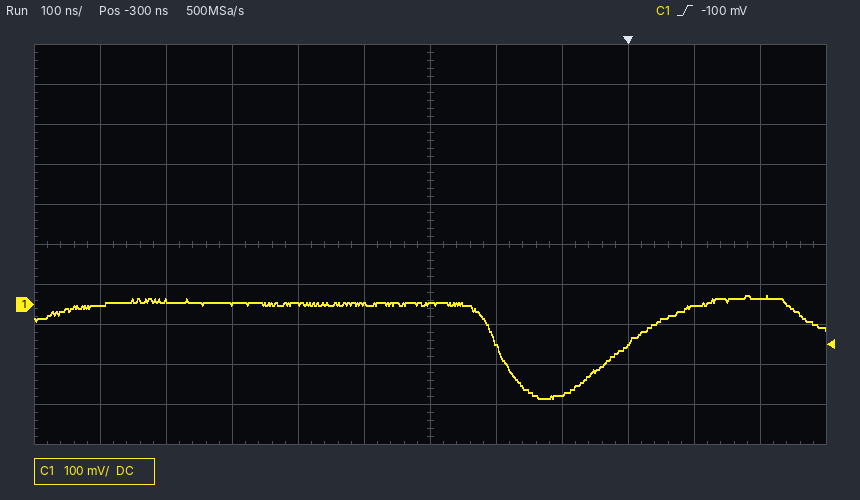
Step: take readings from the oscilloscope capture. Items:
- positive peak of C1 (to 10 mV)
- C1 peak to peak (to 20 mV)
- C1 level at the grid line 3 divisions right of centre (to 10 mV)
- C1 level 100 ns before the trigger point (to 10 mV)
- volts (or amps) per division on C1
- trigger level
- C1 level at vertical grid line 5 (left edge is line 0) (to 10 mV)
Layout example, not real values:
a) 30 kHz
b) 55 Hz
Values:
a) 20 mV
b) 260 mV
c) -100 mV
d) -220 mV
e) 100 mV
f) -100 mV
g) 0 mV
